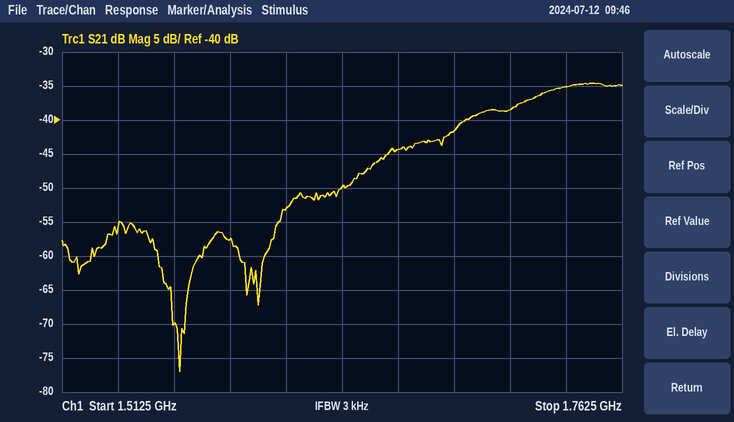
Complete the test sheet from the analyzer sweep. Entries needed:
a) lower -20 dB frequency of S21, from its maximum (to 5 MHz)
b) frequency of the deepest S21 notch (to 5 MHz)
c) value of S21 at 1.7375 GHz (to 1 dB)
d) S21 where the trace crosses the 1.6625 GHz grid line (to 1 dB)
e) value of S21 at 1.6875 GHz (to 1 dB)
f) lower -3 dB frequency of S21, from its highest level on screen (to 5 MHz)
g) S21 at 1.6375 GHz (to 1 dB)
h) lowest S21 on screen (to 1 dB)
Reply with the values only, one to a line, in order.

1.610 GHz
1.565 GHz
-35 dB
-44 dB
-42 dB
1.715 GHz
-50 dB
-77 dB
